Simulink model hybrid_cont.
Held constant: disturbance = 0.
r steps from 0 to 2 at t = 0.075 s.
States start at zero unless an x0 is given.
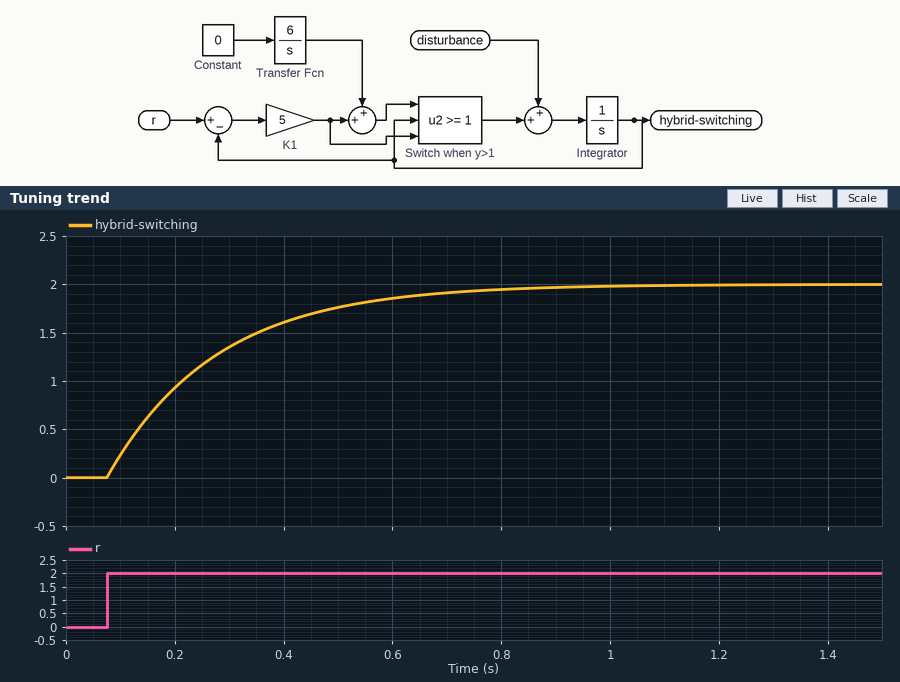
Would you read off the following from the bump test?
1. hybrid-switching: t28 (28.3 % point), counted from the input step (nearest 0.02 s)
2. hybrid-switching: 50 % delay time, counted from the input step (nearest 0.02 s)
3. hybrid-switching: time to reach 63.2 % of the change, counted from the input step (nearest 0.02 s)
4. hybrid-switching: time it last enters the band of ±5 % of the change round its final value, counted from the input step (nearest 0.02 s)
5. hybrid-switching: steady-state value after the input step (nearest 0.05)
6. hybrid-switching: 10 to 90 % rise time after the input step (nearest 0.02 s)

0.06 s
0.14 s
0.20 s
0.60 s
2.00
0.44 s
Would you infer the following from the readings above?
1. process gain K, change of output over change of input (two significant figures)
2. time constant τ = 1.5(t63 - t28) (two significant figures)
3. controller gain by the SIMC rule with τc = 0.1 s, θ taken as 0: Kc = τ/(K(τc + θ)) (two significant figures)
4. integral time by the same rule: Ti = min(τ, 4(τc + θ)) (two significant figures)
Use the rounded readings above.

1.0
0.21 s
2.1
0.21 s
